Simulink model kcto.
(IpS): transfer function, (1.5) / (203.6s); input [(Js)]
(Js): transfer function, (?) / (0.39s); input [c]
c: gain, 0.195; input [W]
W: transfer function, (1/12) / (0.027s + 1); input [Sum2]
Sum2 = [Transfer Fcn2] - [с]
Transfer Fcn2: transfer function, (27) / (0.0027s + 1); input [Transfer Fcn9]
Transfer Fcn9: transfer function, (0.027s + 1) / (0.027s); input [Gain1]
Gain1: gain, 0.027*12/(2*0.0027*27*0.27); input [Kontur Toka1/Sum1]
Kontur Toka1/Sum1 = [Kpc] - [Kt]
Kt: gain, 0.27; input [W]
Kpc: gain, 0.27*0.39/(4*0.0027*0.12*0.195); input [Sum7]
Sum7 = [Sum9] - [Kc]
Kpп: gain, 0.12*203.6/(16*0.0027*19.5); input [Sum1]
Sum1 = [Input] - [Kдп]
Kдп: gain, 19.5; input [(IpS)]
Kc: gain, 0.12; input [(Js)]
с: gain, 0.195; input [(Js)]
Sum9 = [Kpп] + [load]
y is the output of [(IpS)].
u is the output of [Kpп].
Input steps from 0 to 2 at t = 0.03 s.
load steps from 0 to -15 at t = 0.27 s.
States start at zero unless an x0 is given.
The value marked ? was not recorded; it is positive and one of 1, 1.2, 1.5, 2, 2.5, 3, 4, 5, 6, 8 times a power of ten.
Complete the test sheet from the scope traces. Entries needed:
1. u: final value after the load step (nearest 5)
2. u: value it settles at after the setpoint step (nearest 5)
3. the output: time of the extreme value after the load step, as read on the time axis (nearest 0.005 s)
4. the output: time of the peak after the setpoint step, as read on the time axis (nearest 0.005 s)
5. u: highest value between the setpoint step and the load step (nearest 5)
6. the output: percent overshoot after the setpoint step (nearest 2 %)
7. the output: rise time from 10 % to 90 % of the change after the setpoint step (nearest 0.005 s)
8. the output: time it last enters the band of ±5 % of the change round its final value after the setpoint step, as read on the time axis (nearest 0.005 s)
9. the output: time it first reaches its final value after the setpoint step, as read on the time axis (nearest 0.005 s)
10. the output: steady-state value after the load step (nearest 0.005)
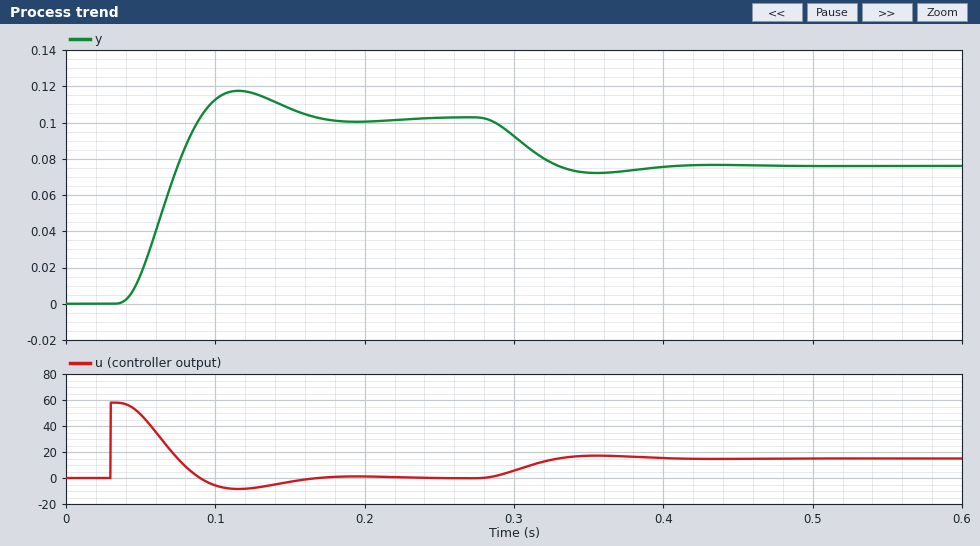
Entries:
15
0
0.355 s
0.115 s
60
14 %
0.035 s
0.150 s
0.090 s
0.075
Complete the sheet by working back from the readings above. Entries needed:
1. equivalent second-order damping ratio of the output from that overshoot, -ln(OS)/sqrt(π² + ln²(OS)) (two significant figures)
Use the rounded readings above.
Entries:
0.53
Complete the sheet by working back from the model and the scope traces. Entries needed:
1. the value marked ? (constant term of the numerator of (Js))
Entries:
0.5
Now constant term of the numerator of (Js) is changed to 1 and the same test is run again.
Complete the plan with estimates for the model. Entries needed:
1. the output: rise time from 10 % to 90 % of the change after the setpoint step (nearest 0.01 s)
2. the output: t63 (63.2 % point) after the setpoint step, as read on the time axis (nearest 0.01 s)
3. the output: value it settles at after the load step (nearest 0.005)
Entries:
0.03 s
0.06 s
0.075
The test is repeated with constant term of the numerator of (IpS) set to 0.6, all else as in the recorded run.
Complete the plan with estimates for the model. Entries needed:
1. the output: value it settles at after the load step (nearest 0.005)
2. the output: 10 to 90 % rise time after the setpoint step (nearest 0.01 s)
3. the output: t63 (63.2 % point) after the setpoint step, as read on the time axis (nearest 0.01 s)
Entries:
0.075
0.11 s
0.11 s
